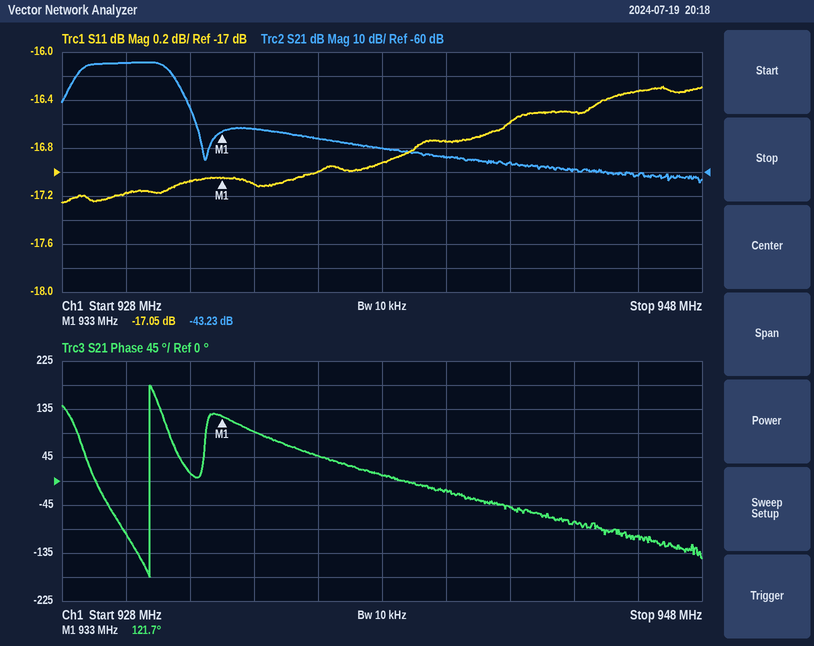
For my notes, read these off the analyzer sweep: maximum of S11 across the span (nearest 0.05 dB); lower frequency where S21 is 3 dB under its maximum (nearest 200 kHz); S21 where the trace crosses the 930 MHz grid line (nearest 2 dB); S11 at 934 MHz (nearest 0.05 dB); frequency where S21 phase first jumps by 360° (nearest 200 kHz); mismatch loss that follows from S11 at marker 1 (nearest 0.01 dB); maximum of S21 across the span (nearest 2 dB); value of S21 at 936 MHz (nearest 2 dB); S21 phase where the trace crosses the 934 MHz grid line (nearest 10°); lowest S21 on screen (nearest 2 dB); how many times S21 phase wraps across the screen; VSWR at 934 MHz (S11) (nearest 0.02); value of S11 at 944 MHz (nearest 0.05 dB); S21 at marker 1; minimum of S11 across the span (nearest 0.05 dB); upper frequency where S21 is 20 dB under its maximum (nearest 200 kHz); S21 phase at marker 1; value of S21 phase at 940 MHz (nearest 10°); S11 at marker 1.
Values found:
-16.30 dB
928.6 MHz
-14 dB
-17.10 dB
930.8 MHz
0.09 dB
-14 dB
-46 dB
90°
-64 dB
1
1.32
-16.50 dB
-43.23 dB
-17.25 dB
932.0 MHz
121.7°
-20°
-17.05 dB
